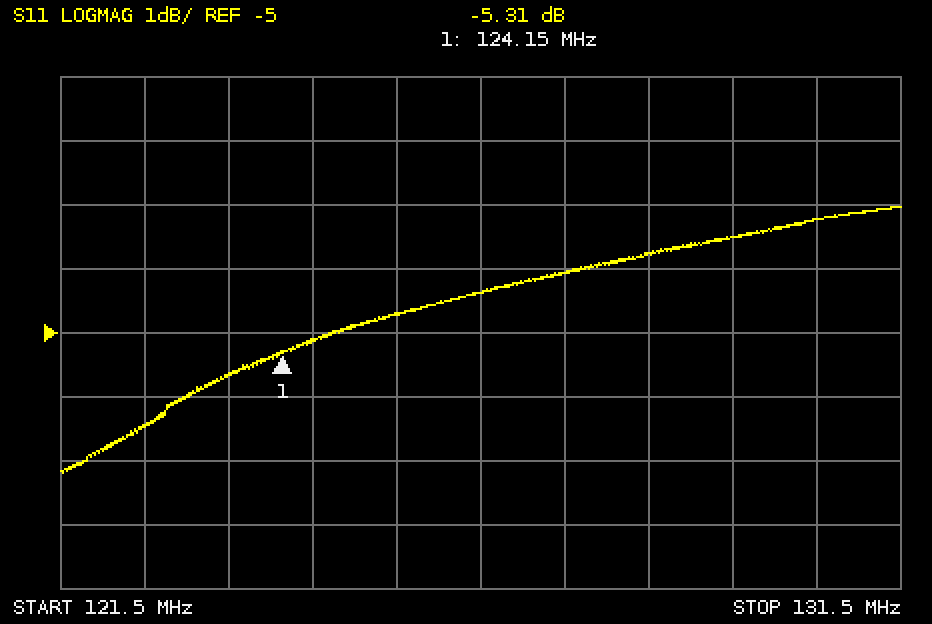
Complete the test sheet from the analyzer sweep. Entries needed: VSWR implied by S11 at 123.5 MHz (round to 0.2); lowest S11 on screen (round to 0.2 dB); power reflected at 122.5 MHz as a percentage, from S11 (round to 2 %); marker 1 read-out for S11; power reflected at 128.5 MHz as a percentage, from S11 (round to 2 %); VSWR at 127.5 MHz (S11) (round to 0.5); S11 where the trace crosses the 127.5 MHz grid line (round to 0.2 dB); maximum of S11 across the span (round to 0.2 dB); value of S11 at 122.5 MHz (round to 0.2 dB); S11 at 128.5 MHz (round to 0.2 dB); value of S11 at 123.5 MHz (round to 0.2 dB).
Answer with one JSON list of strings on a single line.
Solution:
["3.2", "-7.2 dB", "22 %", "-5.31 dB", "42 %", "4.5", "-4.0 dB", "-3.0 dB", "-6.4 dB", "-3.8 dB", "-5.6 dB"]
